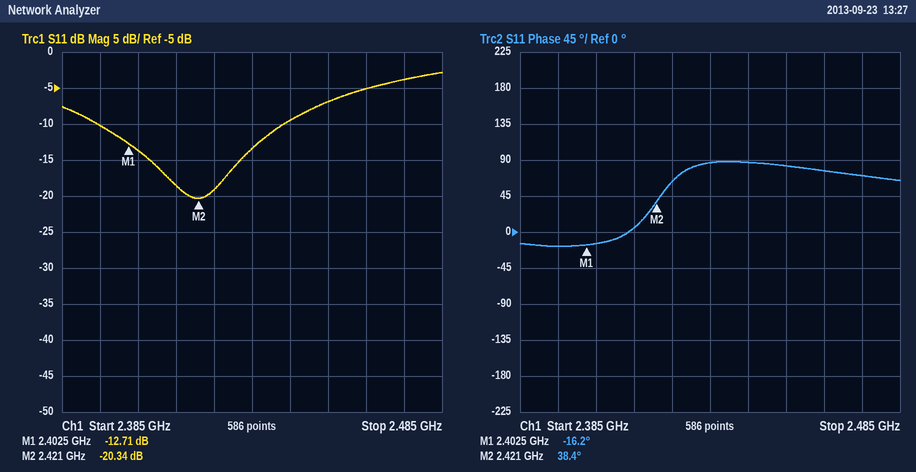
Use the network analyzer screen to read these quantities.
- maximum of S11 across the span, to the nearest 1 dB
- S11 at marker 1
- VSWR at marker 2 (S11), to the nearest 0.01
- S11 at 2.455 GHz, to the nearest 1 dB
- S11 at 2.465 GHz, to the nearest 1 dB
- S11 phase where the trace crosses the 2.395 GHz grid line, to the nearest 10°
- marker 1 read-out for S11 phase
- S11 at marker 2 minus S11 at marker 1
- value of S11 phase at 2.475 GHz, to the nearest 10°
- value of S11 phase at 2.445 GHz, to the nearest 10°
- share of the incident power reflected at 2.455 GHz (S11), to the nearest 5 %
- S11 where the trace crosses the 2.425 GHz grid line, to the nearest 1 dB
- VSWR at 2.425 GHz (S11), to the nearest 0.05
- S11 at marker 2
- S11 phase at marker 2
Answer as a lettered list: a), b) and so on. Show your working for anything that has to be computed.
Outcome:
a) -3 dB
b) -12.71 dB
c) (1 + 0.0962)/(1 − 0.0962) ≈ 1.21
d) -7 dB
e) -5 dB
f) -20°
g) -16.2°
h) -20.34 − (-12.71) = -7.63 dB
i) 70°
j) 90°
k) 10^(-7/10) ≈ 20 %
l) -19 dB
m) |Γ| = 10^(-19/20) = 0.1122; VSWR = (1 + 0.1122)/(1 − 0.1122) ≈ 1.25
n) -20.34 dB
o) 38.4°
